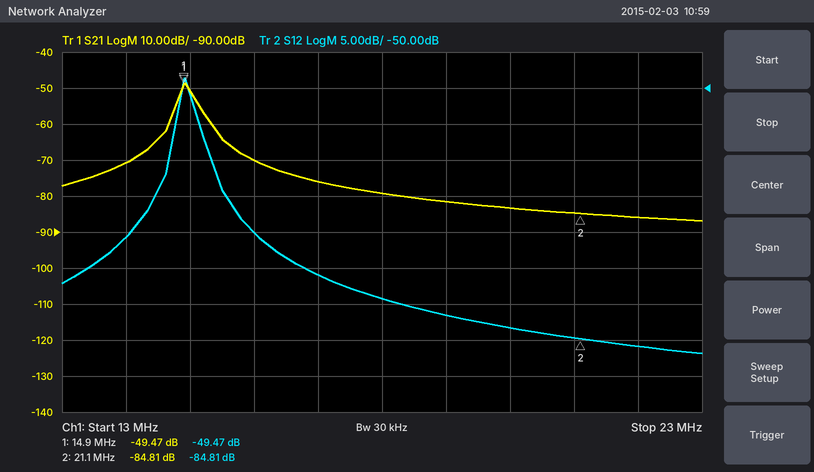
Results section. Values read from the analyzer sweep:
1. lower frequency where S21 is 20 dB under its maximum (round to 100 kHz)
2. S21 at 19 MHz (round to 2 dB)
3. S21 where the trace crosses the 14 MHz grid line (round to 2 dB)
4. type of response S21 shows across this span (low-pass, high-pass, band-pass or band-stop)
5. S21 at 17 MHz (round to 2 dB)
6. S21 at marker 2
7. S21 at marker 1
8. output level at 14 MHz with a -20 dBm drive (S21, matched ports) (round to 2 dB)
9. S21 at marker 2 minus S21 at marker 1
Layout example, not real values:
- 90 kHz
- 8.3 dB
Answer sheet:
- 14.2 MHz
- -82 dB
- -70 dB
- band-pass
- -76 dB
- -84.81 dB
- -49.47 dB
- -90 dBm
- -35.34 dB
